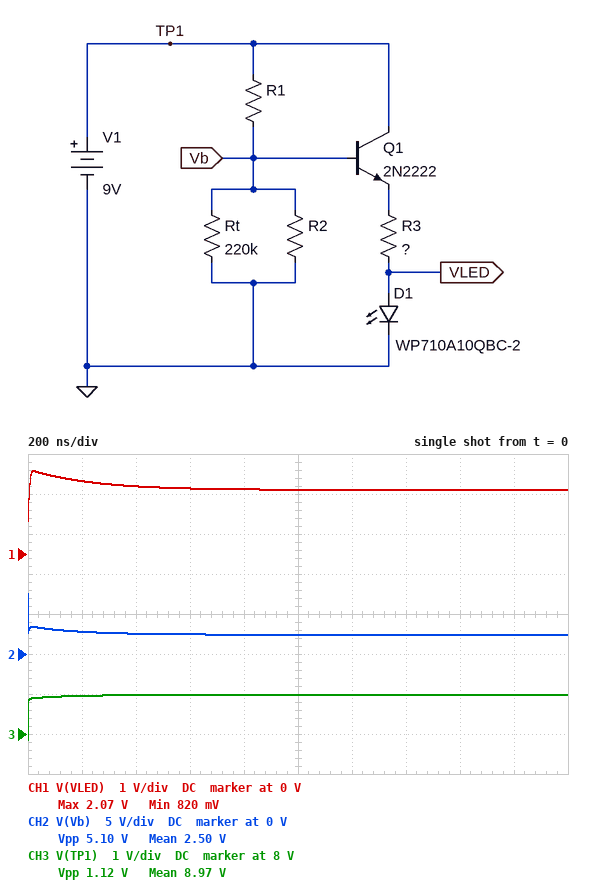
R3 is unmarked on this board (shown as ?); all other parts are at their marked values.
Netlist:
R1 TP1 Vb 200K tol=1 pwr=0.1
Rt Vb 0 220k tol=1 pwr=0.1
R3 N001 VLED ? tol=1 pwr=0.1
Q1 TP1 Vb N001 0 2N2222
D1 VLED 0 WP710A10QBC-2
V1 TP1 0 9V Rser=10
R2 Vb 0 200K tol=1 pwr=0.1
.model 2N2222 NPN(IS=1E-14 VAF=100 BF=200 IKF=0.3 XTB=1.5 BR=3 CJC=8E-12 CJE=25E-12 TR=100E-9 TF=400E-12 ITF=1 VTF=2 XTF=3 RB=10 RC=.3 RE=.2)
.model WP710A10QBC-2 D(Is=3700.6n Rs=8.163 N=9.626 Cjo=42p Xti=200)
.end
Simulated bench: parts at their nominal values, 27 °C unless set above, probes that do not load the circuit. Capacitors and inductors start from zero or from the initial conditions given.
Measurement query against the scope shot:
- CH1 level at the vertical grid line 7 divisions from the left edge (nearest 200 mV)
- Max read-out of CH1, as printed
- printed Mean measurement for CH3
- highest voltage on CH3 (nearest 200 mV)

1.6 V
2.07 V
8.97 V
9.0 V
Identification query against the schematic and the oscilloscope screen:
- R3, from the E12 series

56 Ω
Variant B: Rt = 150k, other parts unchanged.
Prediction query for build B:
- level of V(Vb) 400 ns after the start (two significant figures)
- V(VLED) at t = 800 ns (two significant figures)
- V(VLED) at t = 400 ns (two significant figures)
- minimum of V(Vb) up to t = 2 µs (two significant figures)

2.4 V
1.5 V
1.6 V
2.3 V
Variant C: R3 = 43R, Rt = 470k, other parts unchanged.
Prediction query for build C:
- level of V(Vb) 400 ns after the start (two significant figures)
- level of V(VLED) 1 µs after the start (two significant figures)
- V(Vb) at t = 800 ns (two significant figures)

2.6 V
1.7 V
2.5 V
